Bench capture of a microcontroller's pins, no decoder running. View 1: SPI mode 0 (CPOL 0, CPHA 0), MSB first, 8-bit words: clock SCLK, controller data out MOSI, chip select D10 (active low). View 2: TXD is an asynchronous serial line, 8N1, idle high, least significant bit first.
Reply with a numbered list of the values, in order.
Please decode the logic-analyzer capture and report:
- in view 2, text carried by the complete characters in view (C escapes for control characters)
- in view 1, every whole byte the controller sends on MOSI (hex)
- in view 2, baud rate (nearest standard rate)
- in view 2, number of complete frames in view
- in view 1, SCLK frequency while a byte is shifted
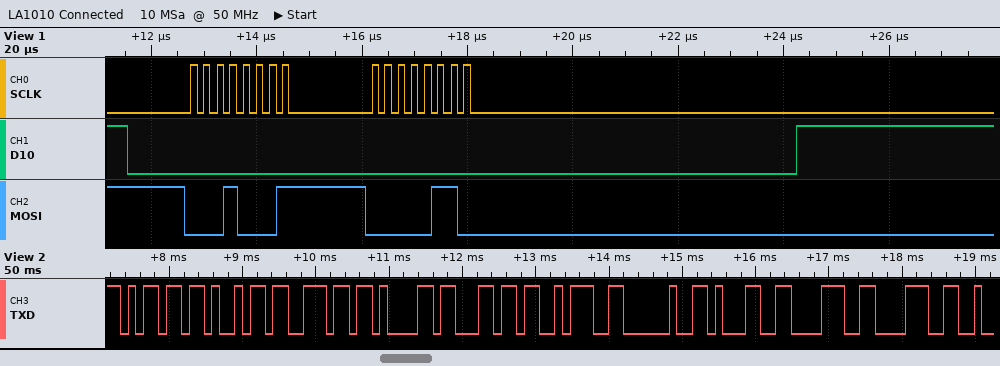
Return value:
1. "minal: 188"
2. 11 06
3. 9600 baud
4. 10
5. 4 MHz
